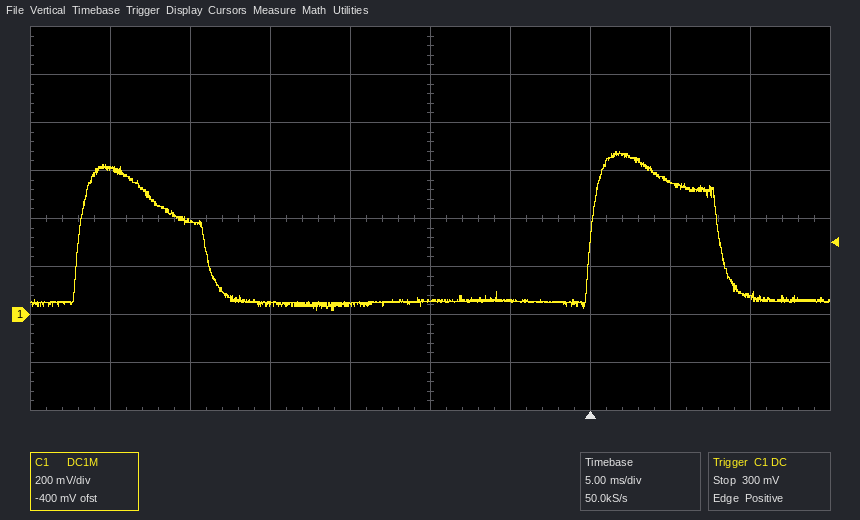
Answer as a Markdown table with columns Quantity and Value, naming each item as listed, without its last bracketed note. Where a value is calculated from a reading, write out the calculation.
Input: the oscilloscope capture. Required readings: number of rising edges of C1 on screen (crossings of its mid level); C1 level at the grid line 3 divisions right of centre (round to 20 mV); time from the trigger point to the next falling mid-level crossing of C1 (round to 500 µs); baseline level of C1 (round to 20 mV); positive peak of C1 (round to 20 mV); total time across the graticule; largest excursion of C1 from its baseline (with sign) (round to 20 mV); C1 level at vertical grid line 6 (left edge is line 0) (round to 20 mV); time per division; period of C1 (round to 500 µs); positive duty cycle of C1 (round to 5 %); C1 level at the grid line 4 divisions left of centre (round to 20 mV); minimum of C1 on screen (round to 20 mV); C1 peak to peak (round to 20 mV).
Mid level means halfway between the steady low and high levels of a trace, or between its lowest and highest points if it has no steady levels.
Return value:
| Quantity | Value |
|---|---|
| number of rising edges of C1 on screen | 2 |
| C1 level at the grid line 3 divisions right of centre | 560 mV |
| time from the trigger point to the next falling mid-level crossing of C1 | 8.0 ms |
| baseline level of C1 | 60 mV |
| positive peak of C1 | 680 mV |
| total time across the graticule | 50 ms |
| largest excursion of C1 from its baseline (with sign) | 680 mV − (60 mV) = +620 mV |
| C1 level at vertical grid line 6 (left edge is line 0) | 60 mV |
| time per division | 5 ms |
| period of C1 | 32.0 ms |
| positive duty cycle of C1 | 25 % |
| C1 level at the grid line 4 divisions left of centre | 600 mV |
| minimum of C1 on screen | 20 mV |
| C1 peak to peak | 680 mV − (20 mV) = 660 mV |
